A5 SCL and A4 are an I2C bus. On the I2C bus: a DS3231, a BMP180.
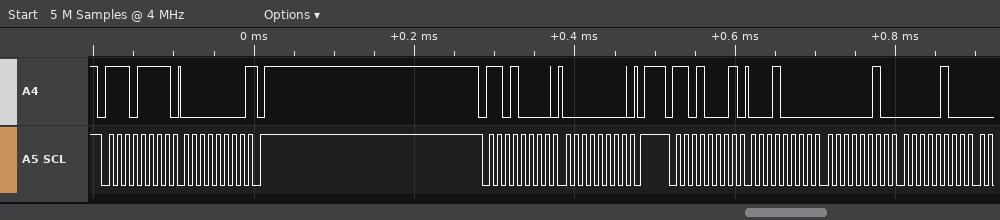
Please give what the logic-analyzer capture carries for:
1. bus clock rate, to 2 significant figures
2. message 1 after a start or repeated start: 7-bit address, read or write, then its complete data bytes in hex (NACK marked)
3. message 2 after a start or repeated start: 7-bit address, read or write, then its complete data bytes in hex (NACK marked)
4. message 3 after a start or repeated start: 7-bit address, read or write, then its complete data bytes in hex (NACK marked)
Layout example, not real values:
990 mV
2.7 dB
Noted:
100 kHz
0x77 read: 00 NACK
0x68 write: 00
0x68 read: 10 02 04
